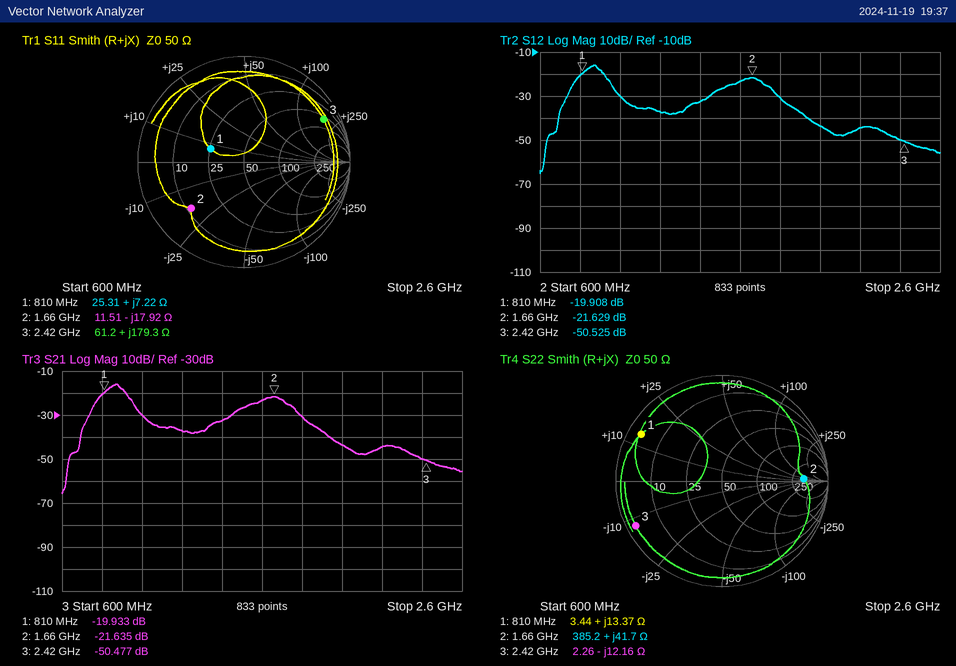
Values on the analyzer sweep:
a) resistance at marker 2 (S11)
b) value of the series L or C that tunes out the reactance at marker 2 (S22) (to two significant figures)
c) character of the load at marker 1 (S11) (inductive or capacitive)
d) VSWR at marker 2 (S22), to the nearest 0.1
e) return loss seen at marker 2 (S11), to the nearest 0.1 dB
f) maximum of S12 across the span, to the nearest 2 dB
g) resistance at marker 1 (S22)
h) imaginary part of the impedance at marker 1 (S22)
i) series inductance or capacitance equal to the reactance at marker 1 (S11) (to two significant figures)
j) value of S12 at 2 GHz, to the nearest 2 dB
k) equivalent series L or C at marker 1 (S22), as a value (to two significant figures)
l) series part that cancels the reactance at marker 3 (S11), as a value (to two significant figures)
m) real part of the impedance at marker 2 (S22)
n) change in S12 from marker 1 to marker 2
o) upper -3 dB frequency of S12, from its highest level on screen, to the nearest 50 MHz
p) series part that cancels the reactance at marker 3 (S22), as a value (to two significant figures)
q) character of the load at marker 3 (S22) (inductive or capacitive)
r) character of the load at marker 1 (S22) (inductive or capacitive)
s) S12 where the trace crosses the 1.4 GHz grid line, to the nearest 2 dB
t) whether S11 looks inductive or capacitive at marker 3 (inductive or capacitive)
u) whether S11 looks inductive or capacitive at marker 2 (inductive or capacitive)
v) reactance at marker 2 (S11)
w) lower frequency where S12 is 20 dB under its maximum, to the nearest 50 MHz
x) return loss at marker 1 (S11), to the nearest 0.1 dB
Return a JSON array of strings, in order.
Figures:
["11.51 Ω", "2.3 pF", "inductive", "7.8", "3.6 dB", "-16 dB", "3.44 Ω", "+13.37 Ω", "1.4 nH", "-44 dB", "2.6 nH", "370 fF", "385.2 Ω", "-1.721 dB", "900 MHz", "800 pH", "capacitive", "inductive", "-32 dB", "inductive", "capacitive", "-17.92 Ω", "700 MHz", "9.4 dB"]
